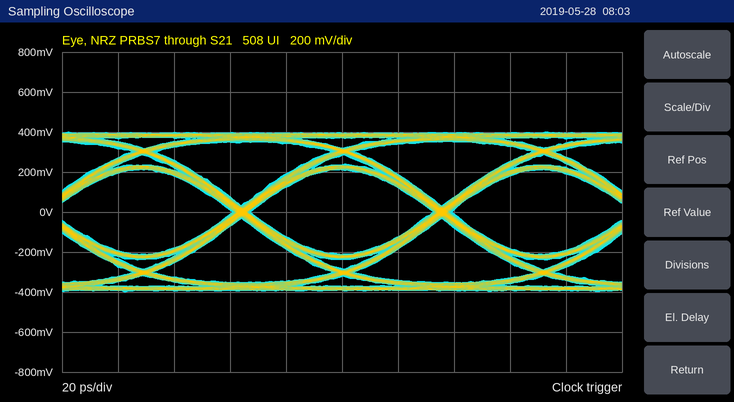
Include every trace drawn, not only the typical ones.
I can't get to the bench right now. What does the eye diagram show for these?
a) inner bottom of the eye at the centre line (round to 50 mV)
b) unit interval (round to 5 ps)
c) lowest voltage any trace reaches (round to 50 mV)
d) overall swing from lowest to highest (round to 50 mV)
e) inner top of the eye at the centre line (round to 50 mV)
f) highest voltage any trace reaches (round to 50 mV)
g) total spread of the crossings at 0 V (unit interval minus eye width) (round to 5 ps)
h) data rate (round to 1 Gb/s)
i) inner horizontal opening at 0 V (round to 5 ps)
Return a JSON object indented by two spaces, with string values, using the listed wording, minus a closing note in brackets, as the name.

{
  "inner bottom of the eye at the centre line": "-200 mV",
  "unit interval": "70 ps",
  "lowest voltage any trace reaches": "-400 mV",
  "overall swing from lowest to highest": "800 mV",
  "inner top of the eye at the centre line": "200 mV",
  "highest voltage any trace reaches": "400 mV",
  "total spread of the crossings at 0 V (unit interval minus eye width)": "5 ps",
  "data rate": "14 Gb/s",
  "inner horizontal opening at 0 V": "65 ps"
}
